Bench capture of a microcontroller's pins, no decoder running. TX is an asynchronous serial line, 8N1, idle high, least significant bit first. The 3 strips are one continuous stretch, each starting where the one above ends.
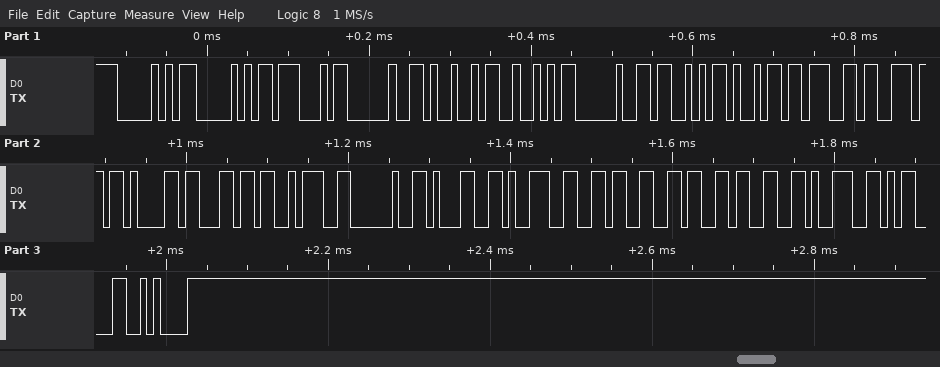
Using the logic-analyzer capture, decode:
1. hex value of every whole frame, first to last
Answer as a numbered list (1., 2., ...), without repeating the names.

1. 50 50 47 20 49 52 20 53 69 67 6E 61 6C 3A 20 31 39 36 36 33 39 0D 0A
